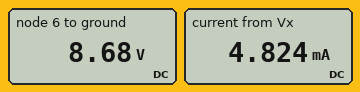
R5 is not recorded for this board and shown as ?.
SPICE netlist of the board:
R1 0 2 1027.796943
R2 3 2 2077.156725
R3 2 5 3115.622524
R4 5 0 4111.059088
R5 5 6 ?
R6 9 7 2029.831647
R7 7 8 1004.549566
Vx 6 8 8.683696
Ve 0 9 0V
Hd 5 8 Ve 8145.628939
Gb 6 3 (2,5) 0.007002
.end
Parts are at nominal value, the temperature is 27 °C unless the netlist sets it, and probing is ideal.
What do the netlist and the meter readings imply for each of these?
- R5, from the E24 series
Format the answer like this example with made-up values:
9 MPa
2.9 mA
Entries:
1.8 kΩ
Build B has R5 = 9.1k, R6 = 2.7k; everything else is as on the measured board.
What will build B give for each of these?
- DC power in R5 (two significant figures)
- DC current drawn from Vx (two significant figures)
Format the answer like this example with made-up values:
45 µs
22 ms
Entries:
8.3 mW
950 µA
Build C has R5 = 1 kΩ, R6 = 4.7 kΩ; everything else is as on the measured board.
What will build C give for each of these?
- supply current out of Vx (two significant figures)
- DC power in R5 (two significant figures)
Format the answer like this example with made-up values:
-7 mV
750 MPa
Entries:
8.7 mA
75 mW
